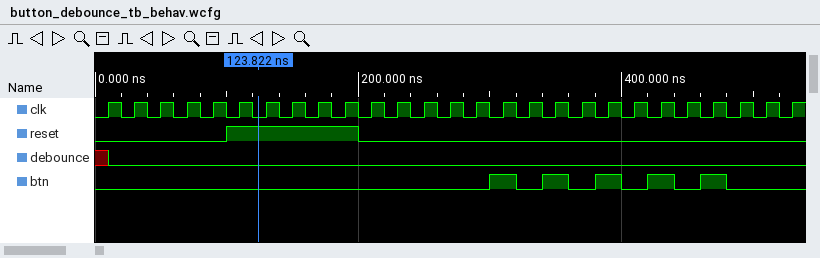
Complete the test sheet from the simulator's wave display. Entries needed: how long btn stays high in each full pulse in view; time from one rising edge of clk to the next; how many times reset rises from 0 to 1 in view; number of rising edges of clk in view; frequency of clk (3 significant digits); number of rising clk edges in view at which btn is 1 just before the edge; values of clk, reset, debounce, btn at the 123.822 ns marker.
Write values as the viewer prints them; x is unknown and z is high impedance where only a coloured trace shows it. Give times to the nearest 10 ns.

20 ns, 20 ns, 20 ns, 20 ns, 20 ns
20 ns
1
27
50.0 MHz
5
clk=0, reset=1, debounce=0, btn=0
